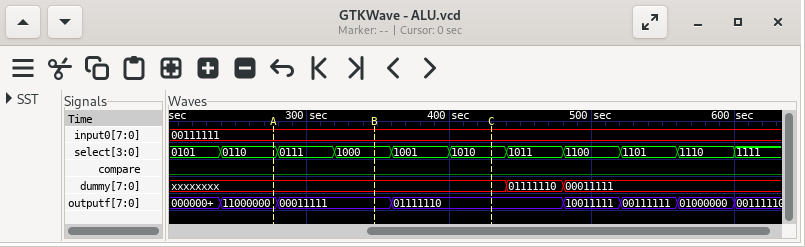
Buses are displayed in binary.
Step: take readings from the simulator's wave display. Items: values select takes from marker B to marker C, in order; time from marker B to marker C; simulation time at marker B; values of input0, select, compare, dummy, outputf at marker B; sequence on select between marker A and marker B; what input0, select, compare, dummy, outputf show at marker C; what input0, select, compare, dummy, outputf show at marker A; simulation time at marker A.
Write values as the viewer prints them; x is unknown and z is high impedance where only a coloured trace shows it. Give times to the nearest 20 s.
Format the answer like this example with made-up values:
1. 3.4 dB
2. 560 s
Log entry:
1. 1000, 1001, 1010
2. 80 s
3. 340 s
4. input0=00111111, select=1000, compare=0, dummy=xxxxxxxx, outputf=00011111
5. 0110, 0111, 1000
6. input0=00111111, select=1010, compare=0, dummy=xxxxxxxx, outputf=01111110
7. input0=00111111, select=0110, compare=0, dummy=xxxxxxxx, outputf=11000000
8. 280 s
